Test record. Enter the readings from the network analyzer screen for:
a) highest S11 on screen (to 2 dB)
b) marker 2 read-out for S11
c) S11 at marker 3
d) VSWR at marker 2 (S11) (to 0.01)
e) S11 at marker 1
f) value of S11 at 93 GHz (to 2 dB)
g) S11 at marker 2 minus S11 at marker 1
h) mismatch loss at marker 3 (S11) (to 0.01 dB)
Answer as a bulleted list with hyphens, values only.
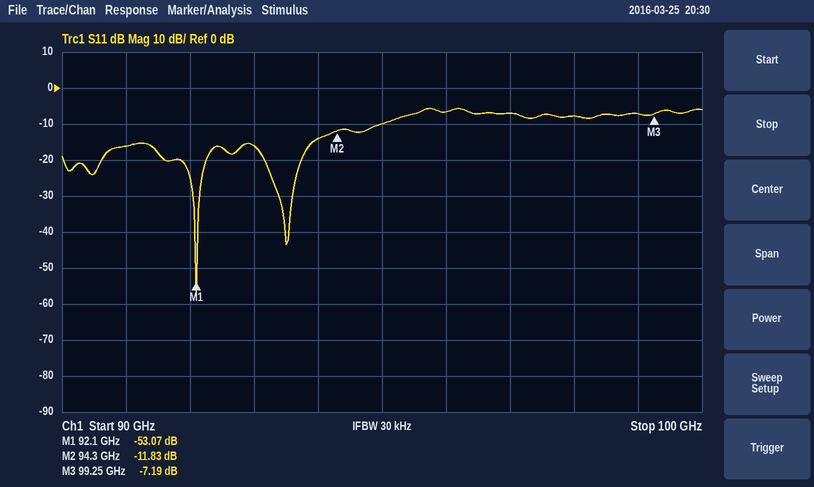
- -6 dB
- -11.83 dB
- -7.19 dB
- 1.69
- -53.07 dB
- -16 dB
- 41.24 dB
- 0.92 dB
